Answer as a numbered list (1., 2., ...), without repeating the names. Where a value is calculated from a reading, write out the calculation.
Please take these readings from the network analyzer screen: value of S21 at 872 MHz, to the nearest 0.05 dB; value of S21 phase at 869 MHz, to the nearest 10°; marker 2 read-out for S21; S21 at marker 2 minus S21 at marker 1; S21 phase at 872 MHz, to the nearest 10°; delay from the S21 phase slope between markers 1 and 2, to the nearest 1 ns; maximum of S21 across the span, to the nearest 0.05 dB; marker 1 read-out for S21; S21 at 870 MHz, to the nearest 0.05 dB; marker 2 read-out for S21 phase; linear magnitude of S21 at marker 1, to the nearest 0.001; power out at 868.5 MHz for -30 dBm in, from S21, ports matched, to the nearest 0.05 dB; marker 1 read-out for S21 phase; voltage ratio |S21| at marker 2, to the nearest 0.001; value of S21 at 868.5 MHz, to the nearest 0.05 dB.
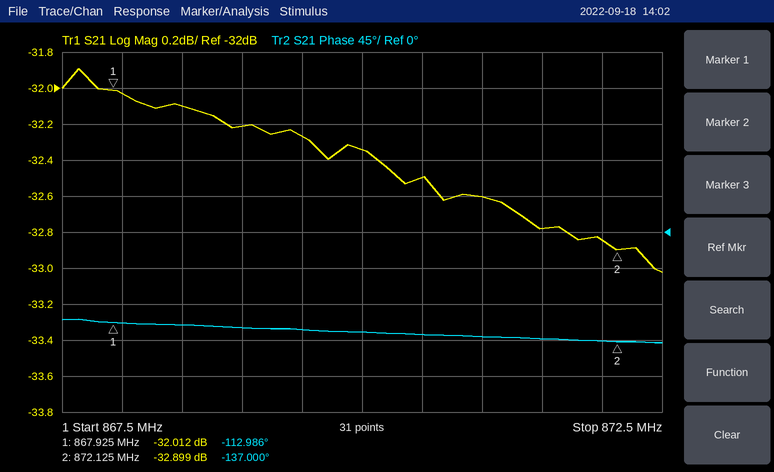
1. -32.85 dB
2. -120°
3. -32.899 dB
4. -32.899 − (-32.012) = -0.887 dB
5. -140°
6. −(-137° − (-112.986°))/(360° × 4.2 MHz) ≈ 16 ns
7. -31.90 dB
8. -32.012 dB
9. -32.35 dB
10. -137.000°
11. 10^(-32.012/20) ≈ 0.025
12. -30 dBm + (-32.10 dB) = -62.10 dBm
13. -112.986°
14. 10^(-32.899/20) ≈ 0.023
15. -32.10 dB
